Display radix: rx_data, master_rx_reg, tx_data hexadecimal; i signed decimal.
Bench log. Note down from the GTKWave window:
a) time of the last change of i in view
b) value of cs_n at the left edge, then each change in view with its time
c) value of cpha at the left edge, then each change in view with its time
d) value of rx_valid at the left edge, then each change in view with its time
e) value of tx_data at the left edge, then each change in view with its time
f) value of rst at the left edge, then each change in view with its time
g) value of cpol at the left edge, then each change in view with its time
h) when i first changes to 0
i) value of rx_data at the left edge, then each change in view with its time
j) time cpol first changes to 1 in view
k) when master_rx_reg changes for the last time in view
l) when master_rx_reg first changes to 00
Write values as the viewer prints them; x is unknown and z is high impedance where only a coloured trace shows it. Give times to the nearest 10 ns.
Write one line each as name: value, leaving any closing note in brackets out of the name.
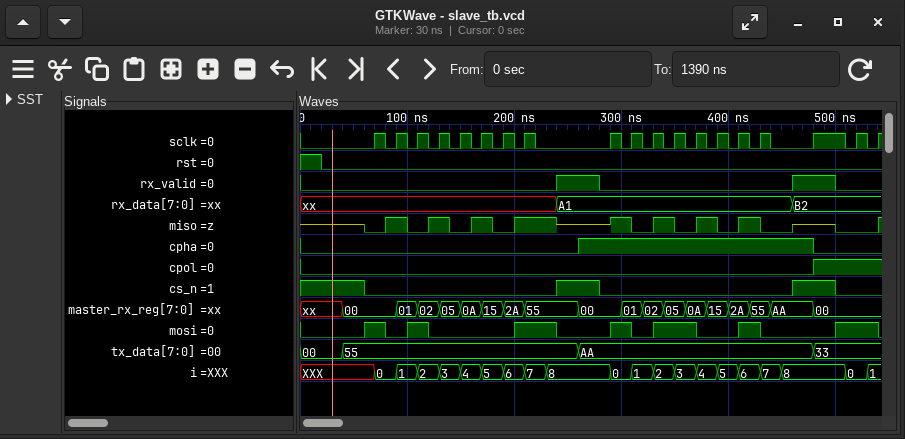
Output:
time of the last change of i in view: 530 ns
value of cs_n at the left edge, then each change in view with its time: 1, 0 at 60 ns, 1 at 240 ns, 0 at 280 ns, 1 at 460 ns, 0 at 500 ns
value of cpha at the left edge, then each change in view with its time: 0, 1 at 260 ns, 0 at 480 ns
value of rx_valid at the left edge, then each change in view with its time: 0, 1 at 240 ns, 0 at 280 ns, 1 at 460 ns, 0 at 500 ns
value of tx_data at the left edge, then each change in view with its time: 00, 55 at 40 ns, AA at 260 ns, 33 at 480 ns
value of rst at the left edge, then each change in view with its time: 1, 0 at 20 ns
value of cpol at the left edge, then each change in view with its time: 0, 1 at 480 ns
when i first changes to 0: 70 ns
value of rx_data at the left edge, then each change in view with its time: xx, A1 at 240 ns, B2 at 460 ns
time cpol first changes to 1 in view: 480 ns
when master_rx_reg changes for the last time in view: 480 ns
when master_rx_reg first changes to 00: 40 ns
